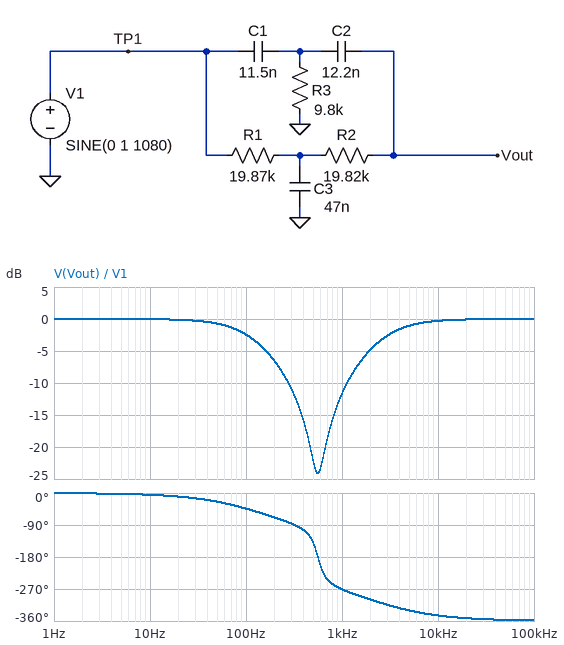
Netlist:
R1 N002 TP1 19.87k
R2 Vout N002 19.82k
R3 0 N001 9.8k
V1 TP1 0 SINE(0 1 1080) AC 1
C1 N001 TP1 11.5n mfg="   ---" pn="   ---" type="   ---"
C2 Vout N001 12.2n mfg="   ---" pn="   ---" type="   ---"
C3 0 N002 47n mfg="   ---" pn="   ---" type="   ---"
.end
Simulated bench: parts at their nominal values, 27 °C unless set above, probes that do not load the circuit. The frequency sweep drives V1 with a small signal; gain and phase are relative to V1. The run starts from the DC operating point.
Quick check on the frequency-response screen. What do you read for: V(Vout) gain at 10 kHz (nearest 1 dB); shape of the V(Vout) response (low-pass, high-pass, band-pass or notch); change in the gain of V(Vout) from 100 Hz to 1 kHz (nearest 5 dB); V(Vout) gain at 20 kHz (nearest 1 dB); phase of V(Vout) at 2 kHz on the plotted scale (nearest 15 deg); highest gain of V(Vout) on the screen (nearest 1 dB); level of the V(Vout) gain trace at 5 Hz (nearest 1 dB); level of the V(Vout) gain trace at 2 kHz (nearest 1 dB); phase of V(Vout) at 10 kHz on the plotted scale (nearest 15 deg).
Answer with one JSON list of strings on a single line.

["0 dB", "notch", "-10 dB", "0 dB", "-300 deg", "0 dB", "0 dB", "-5 dB", "-345 deg"]
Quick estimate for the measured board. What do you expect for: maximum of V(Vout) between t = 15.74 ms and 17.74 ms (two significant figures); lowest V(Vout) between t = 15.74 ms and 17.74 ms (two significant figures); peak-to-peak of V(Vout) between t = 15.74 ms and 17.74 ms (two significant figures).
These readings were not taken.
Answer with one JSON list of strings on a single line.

["300 mV", "-300 mV", "590 mV"]
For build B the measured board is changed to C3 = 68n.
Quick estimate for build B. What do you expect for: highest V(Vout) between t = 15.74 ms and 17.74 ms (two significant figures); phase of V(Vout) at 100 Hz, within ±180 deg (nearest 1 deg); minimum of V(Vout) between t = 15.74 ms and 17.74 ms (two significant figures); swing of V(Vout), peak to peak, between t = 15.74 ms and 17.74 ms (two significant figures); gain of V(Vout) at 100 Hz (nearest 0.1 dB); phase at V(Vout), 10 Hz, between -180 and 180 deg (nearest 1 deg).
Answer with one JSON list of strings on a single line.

["320 mV", "-53 deg", "-320 mV", "650 mV", "-3.5 dB", "-7 deg"]
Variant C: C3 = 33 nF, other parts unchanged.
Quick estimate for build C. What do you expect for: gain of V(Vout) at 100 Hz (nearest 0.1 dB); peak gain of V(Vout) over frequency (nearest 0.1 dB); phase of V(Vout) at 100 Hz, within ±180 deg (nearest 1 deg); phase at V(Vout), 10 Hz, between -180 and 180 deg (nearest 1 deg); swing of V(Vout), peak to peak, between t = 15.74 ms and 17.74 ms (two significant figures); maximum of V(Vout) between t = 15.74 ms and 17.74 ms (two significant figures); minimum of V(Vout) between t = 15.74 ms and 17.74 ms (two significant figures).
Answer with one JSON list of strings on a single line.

["-1.8 dB", "0 dB", "-37 deg", "-4 deg", "530 mV", "260 mV", "-260 mV"]
